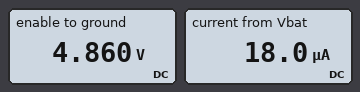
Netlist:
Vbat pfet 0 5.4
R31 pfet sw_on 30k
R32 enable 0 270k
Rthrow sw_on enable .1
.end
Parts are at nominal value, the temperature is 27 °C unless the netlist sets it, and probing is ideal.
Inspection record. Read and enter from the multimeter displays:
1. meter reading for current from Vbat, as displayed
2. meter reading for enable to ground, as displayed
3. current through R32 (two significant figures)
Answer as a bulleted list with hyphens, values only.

- 18.0 µA
- 4.860 V
- 18 µA
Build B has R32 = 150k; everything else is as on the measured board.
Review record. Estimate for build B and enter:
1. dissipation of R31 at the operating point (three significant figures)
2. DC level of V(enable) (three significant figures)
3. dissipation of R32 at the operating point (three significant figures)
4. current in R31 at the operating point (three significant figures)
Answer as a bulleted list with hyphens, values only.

- 27.0 µW
- 4.50 V
- 135 µW
- 30.0 µA
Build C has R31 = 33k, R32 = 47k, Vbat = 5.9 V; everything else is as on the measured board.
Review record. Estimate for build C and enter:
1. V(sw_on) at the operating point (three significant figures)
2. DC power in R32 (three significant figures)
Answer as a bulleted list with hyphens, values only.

- 3.47 V
- 256 µW
